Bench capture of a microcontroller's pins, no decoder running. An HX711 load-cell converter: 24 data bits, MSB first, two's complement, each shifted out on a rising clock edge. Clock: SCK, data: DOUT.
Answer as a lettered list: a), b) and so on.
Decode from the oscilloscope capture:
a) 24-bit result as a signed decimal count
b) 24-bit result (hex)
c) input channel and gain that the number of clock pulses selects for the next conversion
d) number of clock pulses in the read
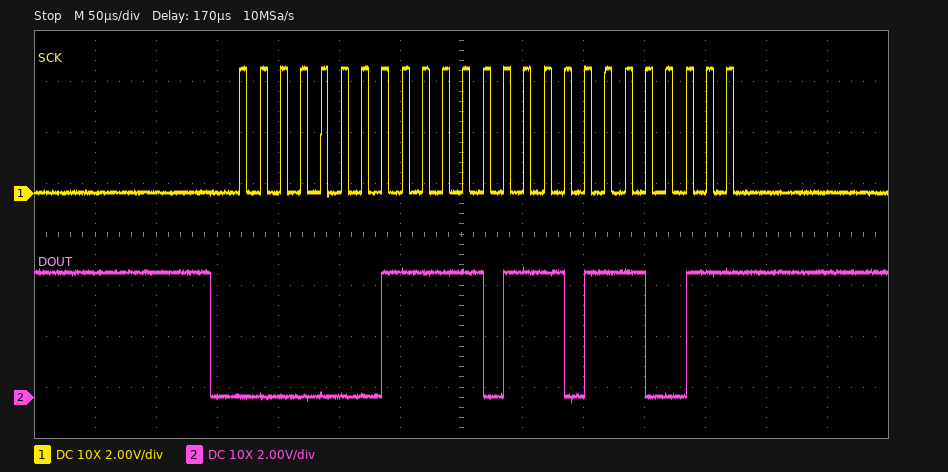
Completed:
a) 128883
b) 0x01F773
c) channel A, gain 128
d) 25
